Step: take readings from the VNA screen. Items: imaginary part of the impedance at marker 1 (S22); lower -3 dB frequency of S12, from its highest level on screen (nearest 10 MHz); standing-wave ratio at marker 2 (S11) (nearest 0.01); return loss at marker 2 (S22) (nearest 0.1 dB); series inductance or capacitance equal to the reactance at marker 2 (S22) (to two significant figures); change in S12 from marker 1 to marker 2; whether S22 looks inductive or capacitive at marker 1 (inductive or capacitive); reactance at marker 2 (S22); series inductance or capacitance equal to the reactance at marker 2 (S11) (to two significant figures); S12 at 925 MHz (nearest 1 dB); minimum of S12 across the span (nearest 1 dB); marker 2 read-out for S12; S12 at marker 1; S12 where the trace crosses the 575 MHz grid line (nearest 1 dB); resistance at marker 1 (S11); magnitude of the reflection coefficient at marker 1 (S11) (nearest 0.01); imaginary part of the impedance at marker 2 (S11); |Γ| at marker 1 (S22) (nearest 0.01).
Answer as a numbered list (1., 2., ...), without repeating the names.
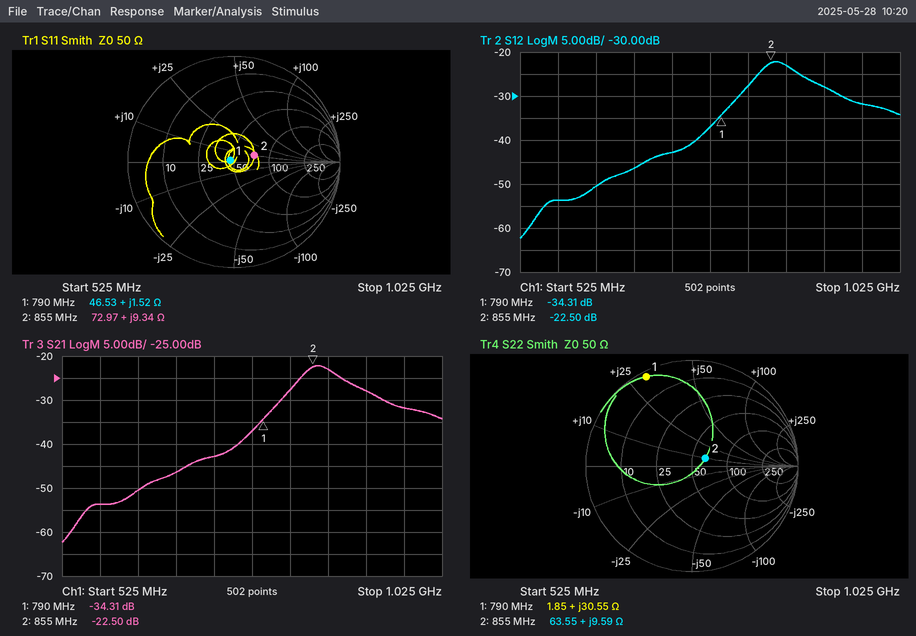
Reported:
1. +30.55 Ω
2. 840 MHz
3. 1.50
4. 16.7 dB
5. 1.8 nH
6. 11.81 dB
7. inductive
8. +9.59 Ω
9. 1.7 nH
10. -28 dB
11. -62 dB
12. -22.50 dB
13. -34.31 dB
14. -54 dB
15. 46.53 Ω
16. 0.04
17. +9.34 Ω
18. 0.95
